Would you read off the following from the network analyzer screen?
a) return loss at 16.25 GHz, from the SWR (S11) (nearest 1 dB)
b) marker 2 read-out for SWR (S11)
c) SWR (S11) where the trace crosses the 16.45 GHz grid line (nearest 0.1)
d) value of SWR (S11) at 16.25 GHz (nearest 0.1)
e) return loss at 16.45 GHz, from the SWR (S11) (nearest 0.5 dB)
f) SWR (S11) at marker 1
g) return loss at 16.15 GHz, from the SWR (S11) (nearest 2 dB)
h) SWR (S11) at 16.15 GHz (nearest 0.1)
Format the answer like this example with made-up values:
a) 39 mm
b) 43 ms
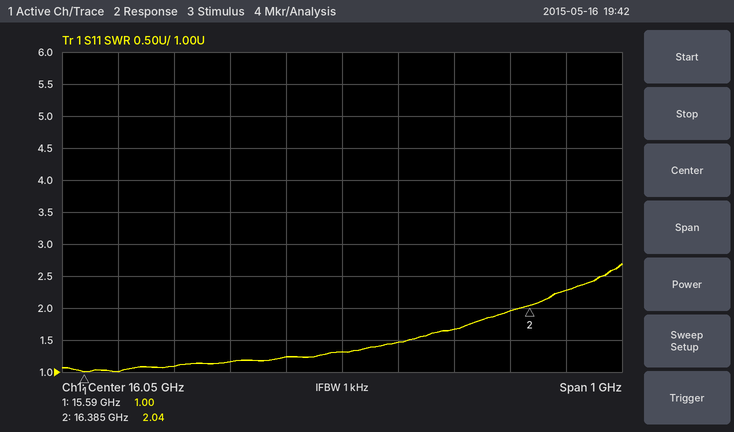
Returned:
a) 12 dB
b) 2.04
c) 2.3
d) 1.7
e) 8.0 dB
f) 1.00
g) 14 dB
h) 1.5
